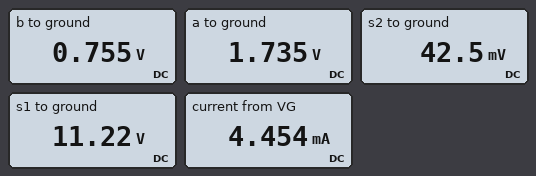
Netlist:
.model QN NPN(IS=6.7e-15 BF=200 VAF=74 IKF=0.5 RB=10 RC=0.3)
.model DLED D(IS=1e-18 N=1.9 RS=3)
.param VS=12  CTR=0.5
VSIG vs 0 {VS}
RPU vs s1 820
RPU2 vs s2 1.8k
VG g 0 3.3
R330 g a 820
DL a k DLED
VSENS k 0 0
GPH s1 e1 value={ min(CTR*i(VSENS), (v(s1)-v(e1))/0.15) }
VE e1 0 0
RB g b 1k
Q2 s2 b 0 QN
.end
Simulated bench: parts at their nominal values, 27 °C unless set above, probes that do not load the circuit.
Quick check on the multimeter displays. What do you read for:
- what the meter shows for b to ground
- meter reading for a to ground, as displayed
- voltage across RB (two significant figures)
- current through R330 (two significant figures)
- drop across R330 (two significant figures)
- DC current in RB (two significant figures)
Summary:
0.755 V
1.735 V
2.5 V
1.9 mA
1.6 V
2.5 mA
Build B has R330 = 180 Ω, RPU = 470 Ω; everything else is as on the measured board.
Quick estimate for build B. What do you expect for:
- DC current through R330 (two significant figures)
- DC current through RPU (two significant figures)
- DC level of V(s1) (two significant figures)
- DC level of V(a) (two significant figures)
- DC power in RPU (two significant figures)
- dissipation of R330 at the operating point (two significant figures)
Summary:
8.2 mA
4.1 mA
10 V
1.8 V
7.9 mW
12 mW
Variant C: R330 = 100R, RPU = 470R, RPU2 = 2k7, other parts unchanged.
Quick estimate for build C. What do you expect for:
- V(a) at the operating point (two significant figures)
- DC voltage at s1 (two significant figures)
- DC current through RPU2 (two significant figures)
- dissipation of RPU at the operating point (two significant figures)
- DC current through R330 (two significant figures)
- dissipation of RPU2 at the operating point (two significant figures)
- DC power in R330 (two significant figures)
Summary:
1.9 V
8.6 V
4.4 mA
24 mW
14 mA
53 mW
20 mW
